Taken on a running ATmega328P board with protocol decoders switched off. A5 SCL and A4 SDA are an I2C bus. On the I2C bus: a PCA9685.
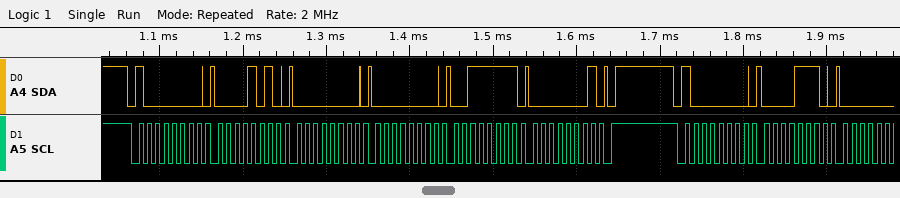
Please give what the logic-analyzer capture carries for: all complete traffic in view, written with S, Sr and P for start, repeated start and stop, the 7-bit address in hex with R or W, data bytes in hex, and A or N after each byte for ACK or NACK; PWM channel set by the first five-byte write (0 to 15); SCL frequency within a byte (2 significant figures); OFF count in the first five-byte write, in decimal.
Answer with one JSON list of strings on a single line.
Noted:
["S 40W A 0A A 00 A 00 A 3F A 01 A P S 40W A 0E A", "1", "100 kHz", "319"]
